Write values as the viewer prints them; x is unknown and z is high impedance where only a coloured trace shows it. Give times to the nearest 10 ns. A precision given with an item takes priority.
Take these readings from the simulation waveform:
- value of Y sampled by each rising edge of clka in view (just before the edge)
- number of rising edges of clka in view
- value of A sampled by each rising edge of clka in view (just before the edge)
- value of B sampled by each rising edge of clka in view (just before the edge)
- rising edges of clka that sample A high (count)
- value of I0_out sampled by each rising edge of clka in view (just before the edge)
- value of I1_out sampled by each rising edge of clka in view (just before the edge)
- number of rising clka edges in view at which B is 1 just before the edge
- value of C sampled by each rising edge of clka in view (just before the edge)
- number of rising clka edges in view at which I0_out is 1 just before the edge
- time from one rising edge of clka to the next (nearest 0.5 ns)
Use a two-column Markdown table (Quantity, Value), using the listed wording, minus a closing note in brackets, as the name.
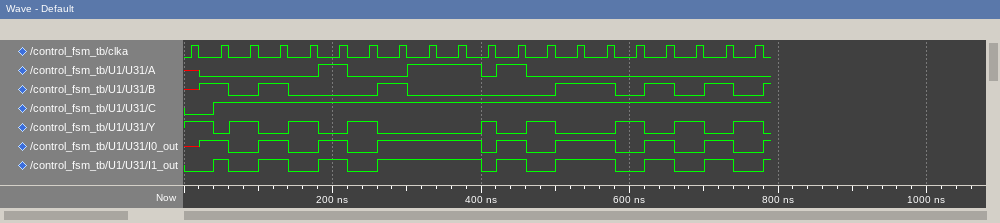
| Quantity | Value |
|---|---|
| value of Y sampled by each rising edge of clka in view | 1 0 1 0 1 0 1 0 0 0 1 0 1 0 0 1 0 1 0 1 |
| number of rising edges of clka in view | 20 |
| value of A sampled by each rising edge of clka in view | x 0 0 0 0 1 0 0 1 1 0 1 0 0 0 0 0 0 0 0 |
| value of B sampled by each rising edge of clka in view | x 1 0 1 0 0 0 1 0 0 0 0 0 1 1 0 1 0 1 0 |
| rising edges of clka that sample A high | 4 |
| value of I0_out sampled by each rising edge of clka in view | x 1 0 1 0 1 0 1 1 1 0 1 0 1 1 0 1 0 1 0 |
| value of I1_out sampled by each rising edge of clka in view | 0 1 0 1 0 1 0 1 1 1 0 1 0 1 1 0 1 0 1 0 |
| number of rising clka edges in view at which B is 1 just before the edge | 7 |
| value of C sampled by each rising edge of clka in view | 0 1 1 1 1 1 1 1 1 1 1 1 1 1 1 1 1 1 1 1 |
| number of rising clka edges in view at which I0_out is 1 just before the edge | 11 |
| time from one rising edge of clka to the next | 40 ns |
